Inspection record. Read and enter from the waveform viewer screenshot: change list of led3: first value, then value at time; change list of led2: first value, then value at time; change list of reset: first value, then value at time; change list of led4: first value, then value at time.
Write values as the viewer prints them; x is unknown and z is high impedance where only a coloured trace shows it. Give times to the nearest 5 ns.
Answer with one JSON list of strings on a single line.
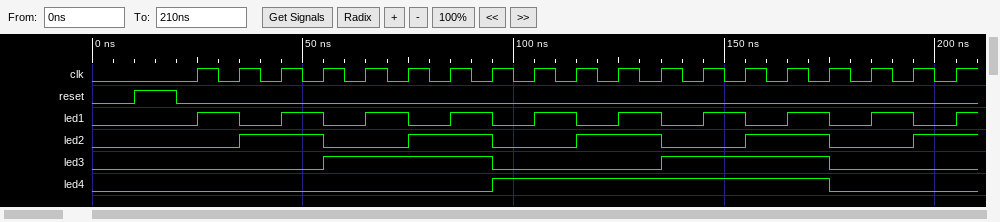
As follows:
["0, 1 at 55 ns, 0 at 95 ns, 1 at 135 ns, 0 at 175 ns", "0, 1 at 35 ns, 0 at 55 ns, 1 at 75 ns, 0 at 95 ns, 1 at 115 ns, 0 at 135 ns, 1 at 155 ns, 0 at 175 ns, 1 at 195 ns", "0, 1 at 10 ns, 0 at 20 ns", "0, 1 at 95 ns, 0 at 175 ns"]
